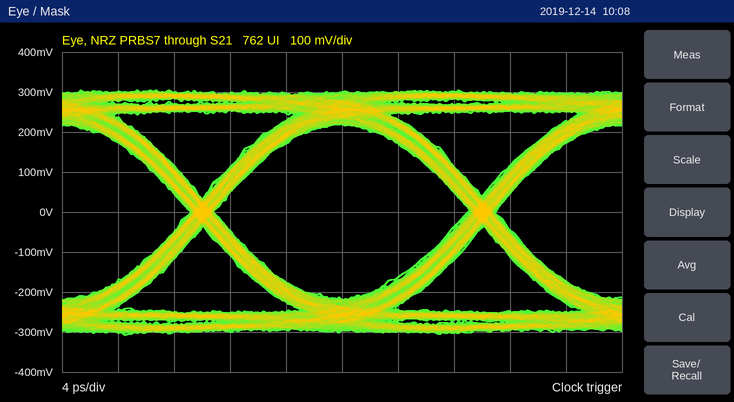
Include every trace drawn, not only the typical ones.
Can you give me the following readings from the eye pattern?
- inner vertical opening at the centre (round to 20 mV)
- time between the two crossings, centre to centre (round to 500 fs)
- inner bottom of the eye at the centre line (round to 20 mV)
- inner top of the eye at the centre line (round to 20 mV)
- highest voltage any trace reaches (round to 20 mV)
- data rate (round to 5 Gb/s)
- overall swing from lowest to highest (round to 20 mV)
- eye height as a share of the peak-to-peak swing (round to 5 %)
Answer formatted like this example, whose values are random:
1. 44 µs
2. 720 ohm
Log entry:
1. 440 mV
2. 20.0 ps
3. -220 mV
4. 220 mV
5. 300 mV
6. 50 Gb/s
7. 620 mV
8. 70 %
